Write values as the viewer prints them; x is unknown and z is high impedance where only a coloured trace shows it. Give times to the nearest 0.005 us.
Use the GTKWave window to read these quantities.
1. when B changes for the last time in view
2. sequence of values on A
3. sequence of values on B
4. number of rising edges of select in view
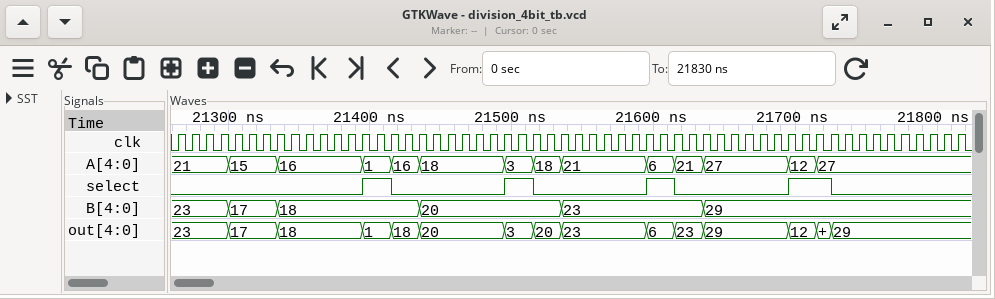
21.635 us
21, 15, 16, 1, 16, 18, 3, 18, 21, 6, 21, 27, 12, 27
23, 17, 18, 20, 23, 29
4
